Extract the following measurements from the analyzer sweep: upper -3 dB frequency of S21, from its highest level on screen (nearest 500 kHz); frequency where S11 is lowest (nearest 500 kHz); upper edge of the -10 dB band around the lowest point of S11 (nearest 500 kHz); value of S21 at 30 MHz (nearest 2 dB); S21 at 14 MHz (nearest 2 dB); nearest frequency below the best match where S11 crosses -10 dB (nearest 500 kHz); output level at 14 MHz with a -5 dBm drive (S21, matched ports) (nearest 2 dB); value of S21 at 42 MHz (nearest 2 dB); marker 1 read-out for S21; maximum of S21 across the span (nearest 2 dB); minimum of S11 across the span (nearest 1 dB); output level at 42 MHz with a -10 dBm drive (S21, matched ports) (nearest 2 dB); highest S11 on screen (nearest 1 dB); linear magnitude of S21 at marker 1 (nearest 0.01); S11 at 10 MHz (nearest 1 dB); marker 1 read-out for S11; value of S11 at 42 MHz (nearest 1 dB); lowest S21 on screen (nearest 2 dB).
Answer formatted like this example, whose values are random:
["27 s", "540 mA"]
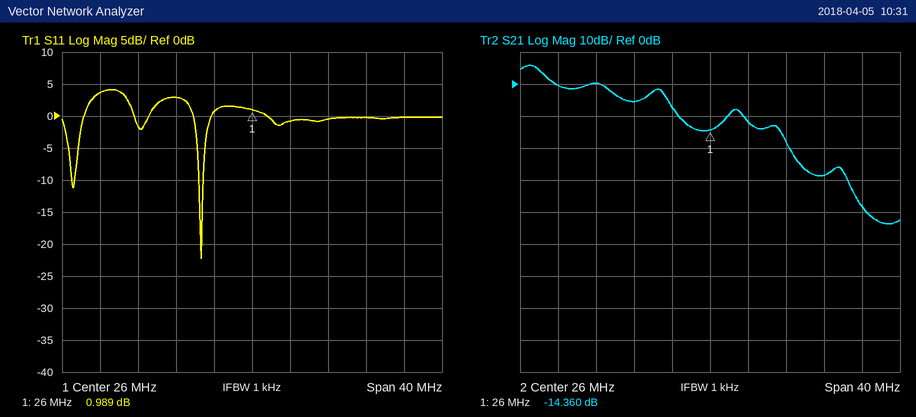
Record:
["8.5 MHz", "20.5 MHz", "21.0 MHz", "-12 dB", "0 dB", "20.5 MHz", "-4 dBm", "-38 dB", "-14.360 dB", "6 dB", "-22 dB", "-48 dBm", "4 dB", "0.19", "4 dB", "0.989 dB", "0 dB", "-44 dB"]
